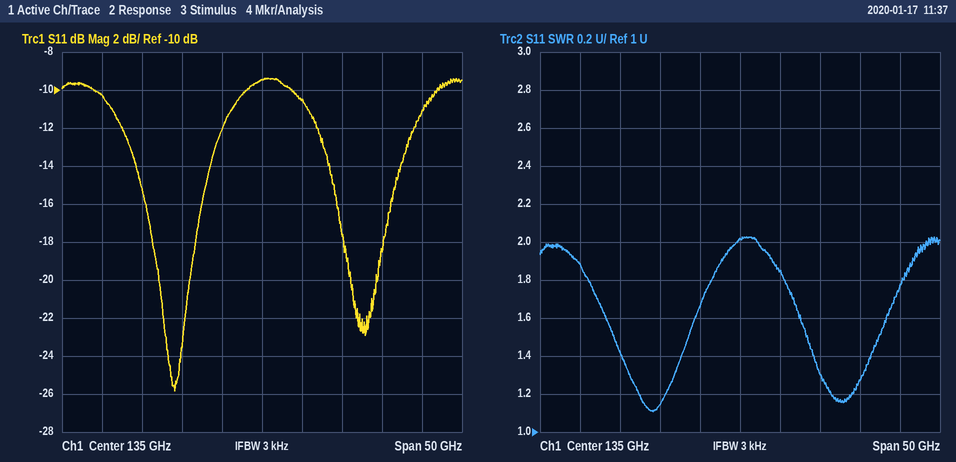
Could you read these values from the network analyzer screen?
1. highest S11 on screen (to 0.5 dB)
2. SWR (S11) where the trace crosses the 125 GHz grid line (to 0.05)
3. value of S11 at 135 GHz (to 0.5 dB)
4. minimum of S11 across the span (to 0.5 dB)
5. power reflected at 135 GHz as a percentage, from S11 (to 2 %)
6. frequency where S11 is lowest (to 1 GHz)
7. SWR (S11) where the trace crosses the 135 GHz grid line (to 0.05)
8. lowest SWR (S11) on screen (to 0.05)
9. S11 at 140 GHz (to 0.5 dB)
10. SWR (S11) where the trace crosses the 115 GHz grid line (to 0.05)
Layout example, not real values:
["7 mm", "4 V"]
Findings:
["-9.5 dB", "1.15", "-9.5 dB", "-26.0 dB", "12 %", "124 GHz", "2.00", "1.10", "-10.5 dB", "1.90"]
